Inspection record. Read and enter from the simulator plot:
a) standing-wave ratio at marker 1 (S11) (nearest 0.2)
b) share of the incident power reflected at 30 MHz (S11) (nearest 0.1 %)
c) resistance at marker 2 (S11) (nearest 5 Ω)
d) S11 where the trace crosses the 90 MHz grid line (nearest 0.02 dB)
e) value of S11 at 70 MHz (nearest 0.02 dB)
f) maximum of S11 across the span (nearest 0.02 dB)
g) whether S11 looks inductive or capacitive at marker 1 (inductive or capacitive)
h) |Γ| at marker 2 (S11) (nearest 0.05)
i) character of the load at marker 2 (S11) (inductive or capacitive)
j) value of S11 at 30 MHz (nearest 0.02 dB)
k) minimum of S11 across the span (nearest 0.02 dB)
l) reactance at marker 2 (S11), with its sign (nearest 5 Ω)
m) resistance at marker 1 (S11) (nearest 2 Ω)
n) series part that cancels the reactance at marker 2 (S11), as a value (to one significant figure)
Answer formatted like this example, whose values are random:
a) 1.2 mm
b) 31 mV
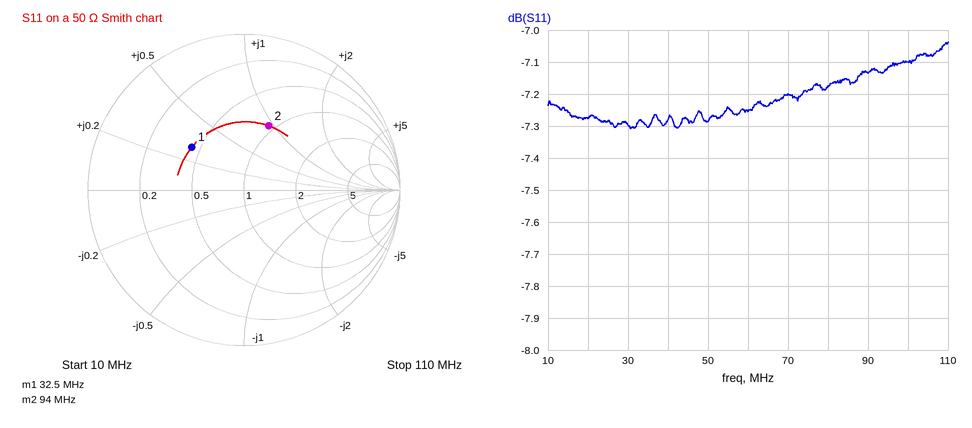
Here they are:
a) 2.6
b) 18.6 %
c) 45 Ω
d) -7.14 dB
e) -7.20 dB
f) -7.04 dB
g) inductive
h) 0.45
i) inductive
j) -7.30 dB
k) -7.30 dB
l) +45 Ω
m) 22 Ω
n) 40 pF
